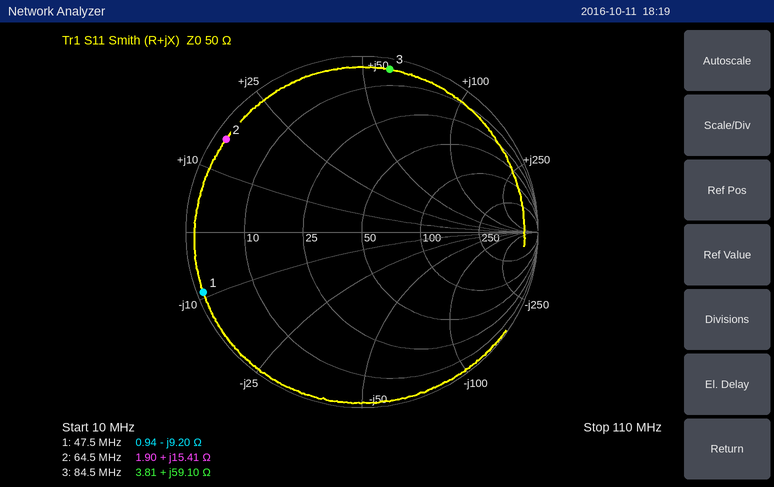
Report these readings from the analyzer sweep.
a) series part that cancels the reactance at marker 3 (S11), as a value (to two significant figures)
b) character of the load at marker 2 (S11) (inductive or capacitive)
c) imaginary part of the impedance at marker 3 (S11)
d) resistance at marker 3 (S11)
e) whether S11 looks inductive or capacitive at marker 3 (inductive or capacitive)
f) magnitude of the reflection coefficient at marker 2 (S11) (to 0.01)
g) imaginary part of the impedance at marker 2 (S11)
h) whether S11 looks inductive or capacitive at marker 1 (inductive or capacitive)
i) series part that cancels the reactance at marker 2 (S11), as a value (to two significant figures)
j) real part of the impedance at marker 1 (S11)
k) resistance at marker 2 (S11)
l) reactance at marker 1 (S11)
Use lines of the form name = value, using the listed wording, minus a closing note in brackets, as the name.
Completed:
series part that cancels the reactance at marker 3 (S11), as a value = 32 pF
character of the load at marker 2 (S11) = inductive
imaginary part of the impedance at marker 3 = +59.10 Ω
resistance at marker 3 = 3.81 Ω
whether S11 looks inductive or capacitive at marker 3 = inductive
magnitude of the reflection coefficient at marker 2 (S11) = 0.93
imaginary part of the impedance at marker 2 = +15.41 Ω
whether S11 looks inductive or capacitive at marker 1 = capacitive
series part that cancels the reactance at marker 2 (S11), as a value = 160 pF
real part of the impedance at marker 1 = 0.94 Ω
resistance at marker 2 = 1.90 Ω
reactance at marker 1 = -9.20 Ω
